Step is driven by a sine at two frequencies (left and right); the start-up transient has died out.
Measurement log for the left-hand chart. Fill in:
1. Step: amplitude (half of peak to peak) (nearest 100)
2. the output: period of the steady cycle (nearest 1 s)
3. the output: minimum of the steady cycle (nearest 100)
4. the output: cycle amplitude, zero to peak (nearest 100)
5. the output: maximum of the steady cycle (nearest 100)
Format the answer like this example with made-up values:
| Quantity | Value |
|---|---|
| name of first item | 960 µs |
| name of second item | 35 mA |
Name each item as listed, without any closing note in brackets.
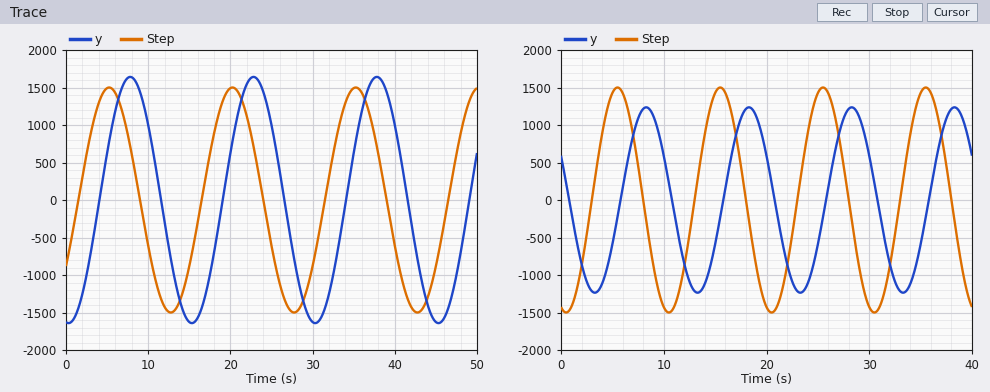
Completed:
| Quantity | Value |
|---|---|
| Step: amplitude (half of peak to peak) | 1500 |
| the output: period of the steady cycle | 15 s |
| the output: minimum of the steady cycle | -1600 |
| the output: cycle amplitude, zero to peak | 1600 |
| the output: maximum of the steady cycle | 1600 |
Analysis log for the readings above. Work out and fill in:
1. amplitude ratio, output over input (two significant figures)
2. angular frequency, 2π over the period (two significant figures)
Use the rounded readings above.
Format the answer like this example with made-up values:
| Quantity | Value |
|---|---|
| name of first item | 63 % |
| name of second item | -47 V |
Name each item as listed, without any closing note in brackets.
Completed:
| Quantity | Value |
|---|---|
| amplitude ratio, output over input | 1.1 |
| angular frequency, 2π over the period | 0.42 rad/s |
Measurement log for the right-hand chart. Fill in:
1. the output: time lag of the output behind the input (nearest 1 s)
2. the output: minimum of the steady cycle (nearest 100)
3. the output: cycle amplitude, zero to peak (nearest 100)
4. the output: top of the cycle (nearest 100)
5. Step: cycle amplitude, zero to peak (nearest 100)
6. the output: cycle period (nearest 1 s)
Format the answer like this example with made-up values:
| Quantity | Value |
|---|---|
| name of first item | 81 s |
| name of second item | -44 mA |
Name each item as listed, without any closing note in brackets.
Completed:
| Quantity | Value |
|---|---|
| the output: time lag of the output behind the input | 3 s |
| the output: minimum of the steady cycle | -1200 |
| the output: cycle amplitude, zero to peak | 1200 |
| the output: top of the cycle | 1200 |
| Step: cycle amplitude, zero to peak | 1500 |
| the output: cycle period | 10 s |
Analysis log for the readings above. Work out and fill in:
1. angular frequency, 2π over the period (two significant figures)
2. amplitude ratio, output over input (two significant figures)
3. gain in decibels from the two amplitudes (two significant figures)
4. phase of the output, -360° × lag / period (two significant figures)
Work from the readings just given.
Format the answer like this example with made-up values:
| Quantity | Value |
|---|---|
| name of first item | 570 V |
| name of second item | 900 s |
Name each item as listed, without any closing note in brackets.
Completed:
| Quantity | Value |
|---|---|
| angular frequency, 2π over the period | 0.63 rad/s |
| amplitude ratio, output over input | 0.80 |
| gain in decibels from the two amplitudes | -1.9 dB |
| phase of the output, -360° × lag / period | -110° |
